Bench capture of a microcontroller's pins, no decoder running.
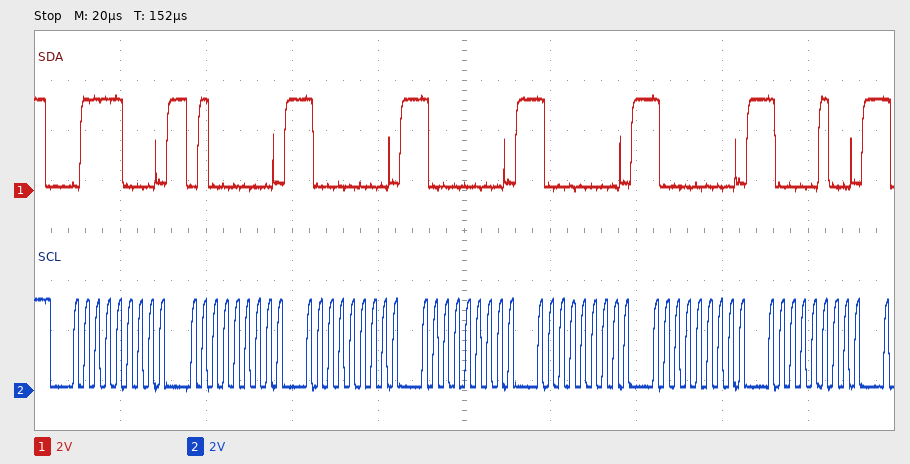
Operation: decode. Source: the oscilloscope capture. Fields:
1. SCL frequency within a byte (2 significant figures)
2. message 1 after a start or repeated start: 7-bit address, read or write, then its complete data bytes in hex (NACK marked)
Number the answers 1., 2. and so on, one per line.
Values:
1. 400 kHz
2. 0x3C write: 40 80 80 80 80 84
